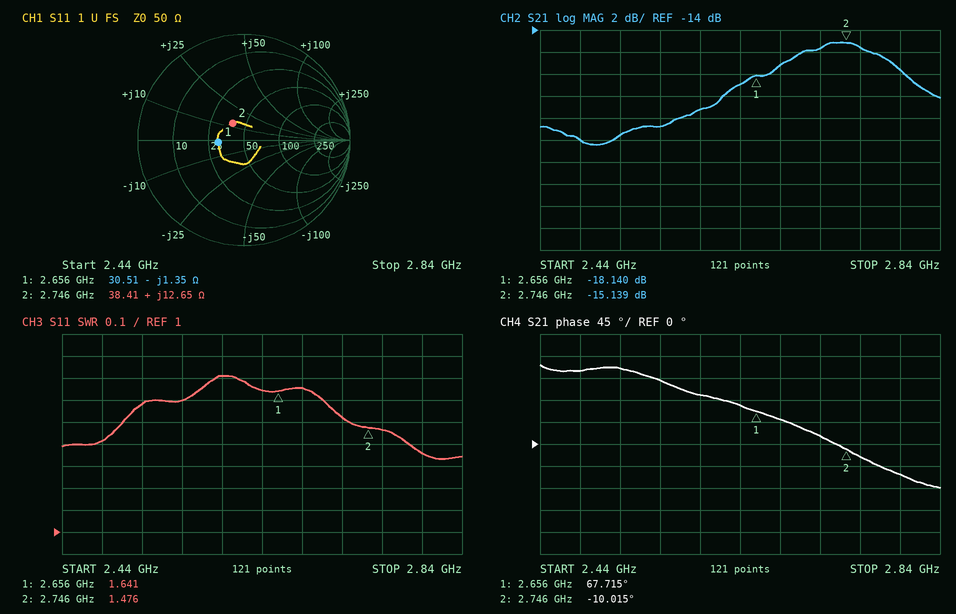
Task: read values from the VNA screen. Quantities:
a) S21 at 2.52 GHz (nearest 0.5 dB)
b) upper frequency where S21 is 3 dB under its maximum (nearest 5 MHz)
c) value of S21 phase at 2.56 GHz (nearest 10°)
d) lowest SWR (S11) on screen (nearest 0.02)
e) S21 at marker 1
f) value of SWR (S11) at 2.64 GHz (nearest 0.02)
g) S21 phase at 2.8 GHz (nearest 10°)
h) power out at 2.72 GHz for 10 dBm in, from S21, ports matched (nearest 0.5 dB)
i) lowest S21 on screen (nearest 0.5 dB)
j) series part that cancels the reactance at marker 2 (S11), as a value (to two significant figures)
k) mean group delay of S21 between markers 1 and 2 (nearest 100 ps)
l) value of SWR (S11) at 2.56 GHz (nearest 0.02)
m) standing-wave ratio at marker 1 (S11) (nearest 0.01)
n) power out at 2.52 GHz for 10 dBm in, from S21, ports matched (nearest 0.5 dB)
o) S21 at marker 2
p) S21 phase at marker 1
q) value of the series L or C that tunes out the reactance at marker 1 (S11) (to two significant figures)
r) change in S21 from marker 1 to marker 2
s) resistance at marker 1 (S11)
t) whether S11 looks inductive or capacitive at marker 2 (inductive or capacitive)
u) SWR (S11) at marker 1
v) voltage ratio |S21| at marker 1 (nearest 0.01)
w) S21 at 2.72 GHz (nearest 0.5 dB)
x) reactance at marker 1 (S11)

-23.5 dB
2.805 GHz
130°
1.34
-18.140 dB
1.64
-60°
-5.5 dBm
-24.5 dB
4.6 pF
2.4 ns
1.60
1.64
-13.5 dBm
-15.139 dB
67.715°
81 pH
3.001 dB
30.51 Ω
inductive
1.641
0.12
-15.5 dB
-1.35 Ω
